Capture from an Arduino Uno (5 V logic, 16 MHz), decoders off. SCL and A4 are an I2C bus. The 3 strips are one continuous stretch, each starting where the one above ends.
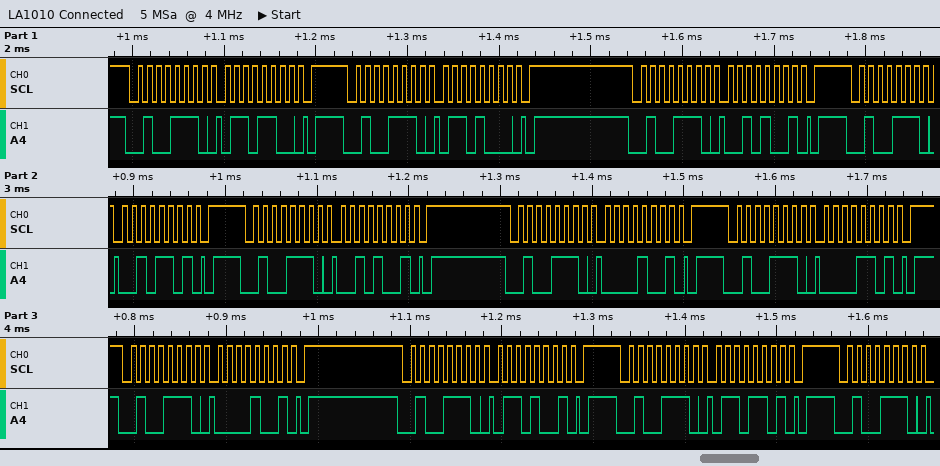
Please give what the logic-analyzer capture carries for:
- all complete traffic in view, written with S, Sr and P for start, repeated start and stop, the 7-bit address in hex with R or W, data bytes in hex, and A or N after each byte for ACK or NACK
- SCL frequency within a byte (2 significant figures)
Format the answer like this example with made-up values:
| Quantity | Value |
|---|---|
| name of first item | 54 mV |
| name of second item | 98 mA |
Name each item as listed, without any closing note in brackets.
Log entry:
| Quantity | Value |
|---|---|
| all complete traffic in view, written with S, Sr and P for start, repeated start and stop, the 7-bit address in hex with R or W, data bytes in hex, and A or N after each byte for ACK or NACK | S 27W A 6C A P S 27W A 68 A P S 27W A 29 A P S 27W A 2D A P S 27W A 29 A P S 27W A 09 A P S 27W A 0D A P S 27W A 09 A P S 27W A 69 A P S 27W A 6D A P S 27W A |
| SCL frequency within a byte | 100 kHz |
